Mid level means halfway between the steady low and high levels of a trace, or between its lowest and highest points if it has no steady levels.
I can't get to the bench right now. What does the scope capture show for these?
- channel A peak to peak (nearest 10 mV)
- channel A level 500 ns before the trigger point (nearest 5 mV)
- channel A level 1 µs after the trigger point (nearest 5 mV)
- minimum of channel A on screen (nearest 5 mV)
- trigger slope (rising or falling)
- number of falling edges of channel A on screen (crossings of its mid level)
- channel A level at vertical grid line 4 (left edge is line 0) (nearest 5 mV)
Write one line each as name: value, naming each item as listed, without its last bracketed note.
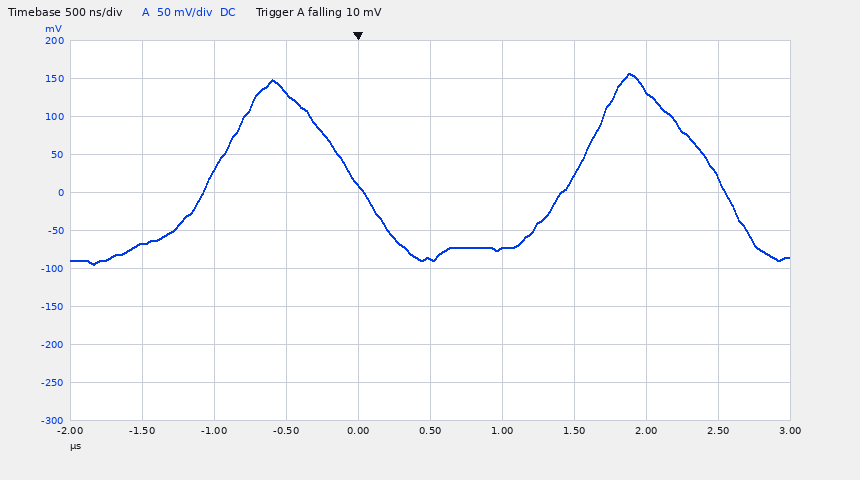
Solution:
channel A peak to peak: 250 mV
channel A level 500 ns before the trigger point: 130 mV
channel A level 1 µs after the trigger point: -75 mV
minimum of channel A on screen: -95 mV
trigger slope: falling
number of falling edges of channel A on screen: 2
channel A level at vertical grid line 4 (left edge is line 0): 10 mV
